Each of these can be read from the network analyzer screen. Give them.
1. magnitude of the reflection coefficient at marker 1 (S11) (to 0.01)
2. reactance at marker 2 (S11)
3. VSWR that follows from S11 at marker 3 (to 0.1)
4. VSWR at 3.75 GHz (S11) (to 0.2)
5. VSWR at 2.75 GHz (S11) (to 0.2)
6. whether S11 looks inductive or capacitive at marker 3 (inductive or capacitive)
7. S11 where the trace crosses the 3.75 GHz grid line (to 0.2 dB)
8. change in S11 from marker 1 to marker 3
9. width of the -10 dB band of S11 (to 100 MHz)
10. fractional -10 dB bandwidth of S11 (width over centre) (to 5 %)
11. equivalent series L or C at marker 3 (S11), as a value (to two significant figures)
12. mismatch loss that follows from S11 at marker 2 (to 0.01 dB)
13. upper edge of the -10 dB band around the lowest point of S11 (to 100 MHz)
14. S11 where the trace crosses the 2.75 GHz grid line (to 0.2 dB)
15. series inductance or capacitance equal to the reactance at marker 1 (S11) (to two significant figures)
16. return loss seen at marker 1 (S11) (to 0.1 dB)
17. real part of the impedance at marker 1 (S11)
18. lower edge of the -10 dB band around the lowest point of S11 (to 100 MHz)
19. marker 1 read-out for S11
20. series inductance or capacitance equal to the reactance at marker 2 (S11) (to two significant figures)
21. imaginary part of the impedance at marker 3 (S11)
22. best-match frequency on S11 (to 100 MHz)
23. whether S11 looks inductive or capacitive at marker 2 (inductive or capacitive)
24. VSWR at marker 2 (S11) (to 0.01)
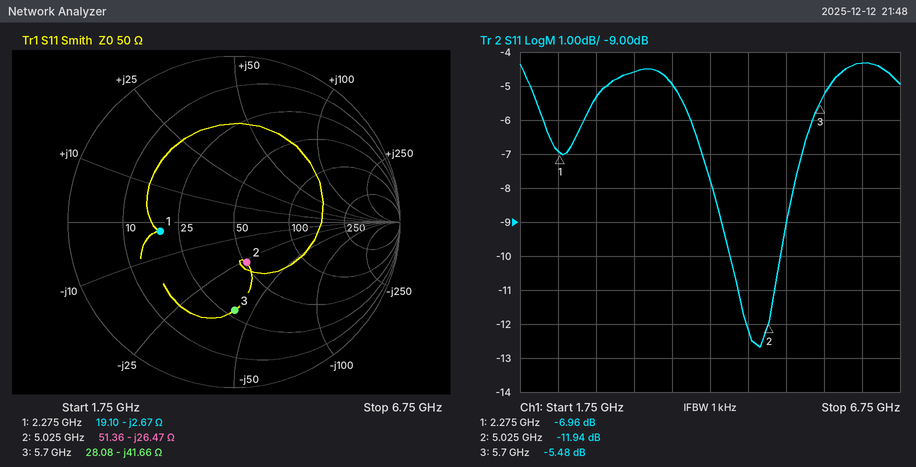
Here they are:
0.45
-26.47 Ω
3.3
3.6
3.4
capacitive
-5.0 dB
1.48 dB
700 MHz
15 %
670 fF
0.29 dB
5.2 GHz
-5.4 dB
26 pF
7.0 dB
19.10 Ω
4.5 GHz
-6.96 dB
1.2 pF
-41.66 Ω
4.9 GHz
capacitive
1.68
